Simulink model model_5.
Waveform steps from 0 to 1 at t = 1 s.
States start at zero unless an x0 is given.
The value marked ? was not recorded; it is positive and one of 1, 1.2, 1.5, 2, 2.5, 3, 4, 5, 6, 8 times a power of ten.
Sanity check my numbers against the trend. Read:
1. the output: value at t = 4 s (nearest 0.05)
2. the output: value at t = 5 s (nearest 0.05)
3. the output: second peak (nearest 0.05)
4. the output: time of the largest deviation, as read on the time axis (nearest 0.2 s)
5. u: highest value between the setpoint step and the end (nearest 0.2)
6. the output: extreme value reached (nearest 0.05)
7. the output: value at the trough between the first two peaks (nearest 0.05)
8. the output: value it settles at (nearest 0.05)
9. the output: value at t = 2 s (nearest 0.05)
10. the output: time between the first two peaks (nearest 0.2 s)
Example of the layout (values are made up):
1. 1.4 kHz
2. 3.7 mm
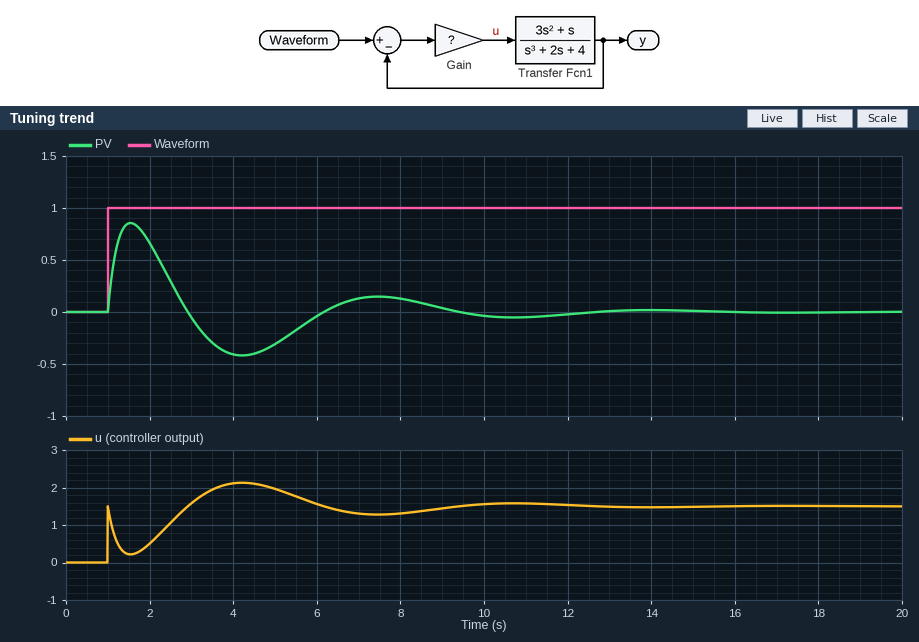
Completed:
1. -0.40
2. -0.30
3. 0.15
4. 1.6 s
5. 2.2
6. 0.85
7. -0.40
8. 0.00
9. 0.65
10. 6.0 s
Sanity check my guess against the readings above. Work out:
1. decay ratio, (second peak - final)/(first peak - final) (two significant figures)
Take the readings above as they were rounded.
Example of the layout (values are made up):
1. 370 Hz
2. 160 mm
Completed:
1. 0.18
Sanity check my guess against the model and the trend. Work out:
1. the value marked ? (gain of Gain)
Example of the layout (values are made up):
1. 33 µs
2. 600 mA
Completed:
1. 1.5
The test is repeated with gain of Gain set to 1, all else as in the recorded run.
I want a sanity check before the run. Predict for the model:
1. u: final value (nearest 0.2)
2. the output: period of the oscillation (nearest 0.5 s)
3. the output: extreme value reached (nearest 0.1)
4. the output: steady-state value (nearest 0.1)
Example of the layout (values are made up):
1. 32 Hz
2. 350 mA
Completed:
1. 1.0
2. 4.5 s
3. 0.8
4. 0.0
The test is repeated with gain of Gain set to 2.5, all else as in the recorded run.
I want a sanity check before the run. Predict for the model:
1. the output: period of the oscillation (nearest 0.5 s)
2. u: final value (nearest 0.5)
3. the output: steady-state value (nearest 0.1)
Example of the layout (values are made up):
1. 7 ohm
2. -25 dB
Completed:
1. 8.0 s
2. 2.5
3. 0.0
